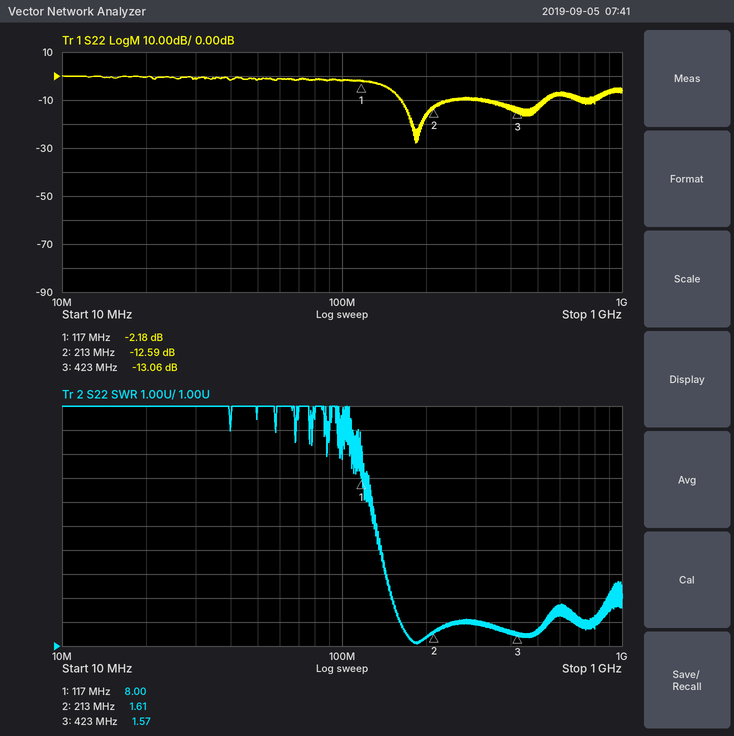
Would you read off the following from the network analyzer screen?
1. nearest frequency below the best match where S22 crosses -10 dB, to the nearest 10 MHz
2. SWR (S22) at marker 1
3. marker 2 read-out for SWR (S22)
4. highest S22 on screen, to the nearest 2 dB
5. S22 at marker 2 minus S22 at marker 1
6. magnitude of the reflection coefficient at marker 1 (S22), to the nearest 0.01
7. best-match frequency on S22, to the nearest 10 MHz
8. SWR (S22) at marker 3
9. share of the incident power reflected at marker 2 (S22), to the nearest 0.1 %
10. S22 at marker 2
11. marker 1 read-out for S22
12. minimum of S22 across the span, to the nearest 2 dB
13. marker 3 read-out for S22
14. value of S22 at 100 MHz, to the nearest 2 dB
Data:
160 MHz
8.00
1.61
0 dB
-10.41 dB
0.78
180 MHz
1.57
5.5 %
-12.59 dB
-2.18 dB
-28 dB
-13.06 dB
-2 dB
